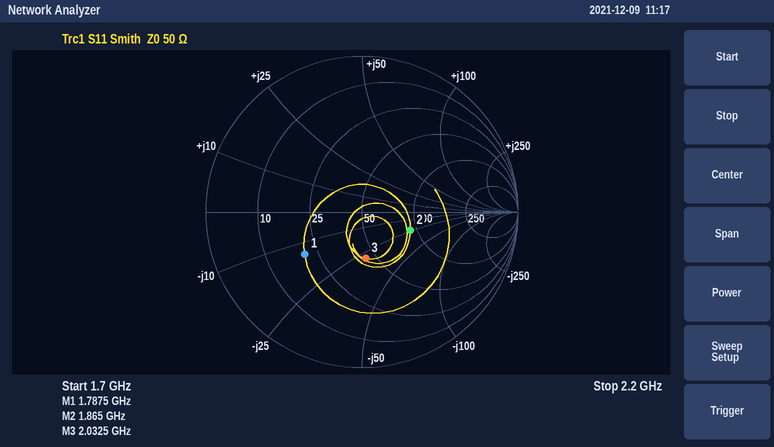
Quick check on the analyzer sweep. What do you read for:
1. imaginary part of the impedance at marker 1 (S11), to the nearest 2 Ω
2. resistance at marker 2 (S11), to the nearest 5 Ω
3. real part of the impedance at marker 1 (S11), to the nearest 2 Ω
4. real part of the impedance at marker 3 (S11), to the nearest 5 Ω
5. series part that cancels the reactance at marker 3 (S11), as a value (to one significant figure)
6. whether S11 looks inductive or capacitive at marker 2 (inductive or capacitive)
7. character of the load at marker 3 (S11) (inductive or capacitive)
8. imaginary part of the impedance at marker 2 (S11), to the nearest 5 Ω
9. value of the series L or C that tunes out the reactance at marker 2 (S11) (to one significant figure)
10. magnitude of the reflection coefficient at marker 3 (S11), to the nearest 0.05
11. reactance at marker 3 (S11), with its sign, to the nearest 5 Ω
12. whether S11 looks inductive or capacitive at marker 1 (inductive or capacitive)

-14 Ω
90 Ω
20 Ω
45 Ω
2 nH
capacitive
capacitive
-25 Ω
2 nH
0.30
-30 Ω
capacitive
